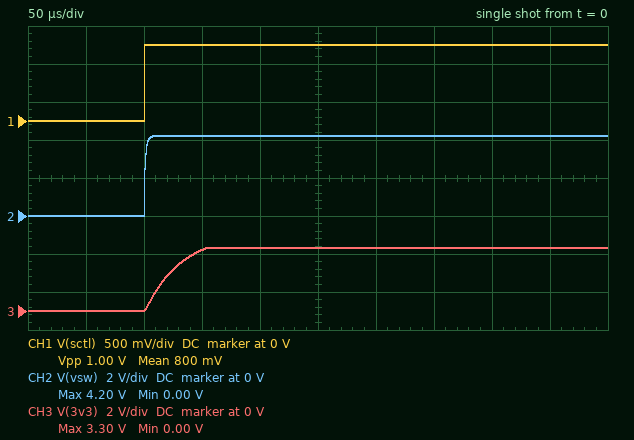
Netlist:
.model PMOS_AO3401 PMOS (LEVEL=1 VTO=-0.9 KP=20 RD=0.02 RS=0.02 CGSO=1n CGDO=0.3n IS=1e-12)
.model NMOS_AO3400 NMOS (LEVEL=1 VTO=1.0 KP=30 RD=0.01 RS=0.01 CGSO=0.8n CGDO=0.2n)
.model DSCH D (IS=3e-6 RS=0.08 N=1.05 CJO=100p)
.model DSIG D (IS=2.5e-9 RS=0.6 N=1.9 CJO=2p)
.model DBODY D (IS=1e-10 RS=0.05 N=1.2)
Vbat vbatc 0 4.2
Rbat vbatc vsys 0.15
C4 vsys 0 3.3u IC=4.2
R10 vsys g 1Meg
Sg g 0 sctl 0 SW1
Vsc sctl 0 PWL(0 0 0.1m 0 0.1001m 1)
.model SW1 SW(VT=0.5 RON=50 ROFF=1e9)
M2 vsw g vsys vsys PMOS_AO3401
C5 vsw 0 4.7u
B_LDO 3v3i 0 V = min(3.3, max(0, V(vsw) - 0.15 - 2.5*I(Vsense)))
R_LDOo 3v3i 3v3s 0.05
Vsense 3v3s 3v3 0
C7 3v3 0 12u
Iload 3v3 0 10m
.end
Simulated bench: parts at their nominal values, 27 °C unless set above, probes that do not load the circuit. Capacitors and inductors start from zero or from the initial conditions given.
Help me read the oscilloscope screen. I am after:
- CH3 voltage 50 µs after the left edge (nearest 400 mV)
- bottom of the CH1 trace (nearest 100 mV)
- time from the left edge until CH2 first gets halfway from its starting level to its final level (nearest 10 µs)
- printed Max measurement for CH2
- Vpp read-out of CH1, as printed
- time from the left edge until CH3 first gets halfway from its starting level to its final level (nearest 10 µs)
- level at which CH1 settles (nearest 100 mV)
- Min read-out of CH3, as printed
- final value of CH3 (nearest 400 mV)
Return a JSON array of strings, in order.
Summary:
["0 V", "0 V", "100 µs", "4.20 V", "1.00 V", "120 µs", "1.0 V", "0.00 V", "3.2 V"]
